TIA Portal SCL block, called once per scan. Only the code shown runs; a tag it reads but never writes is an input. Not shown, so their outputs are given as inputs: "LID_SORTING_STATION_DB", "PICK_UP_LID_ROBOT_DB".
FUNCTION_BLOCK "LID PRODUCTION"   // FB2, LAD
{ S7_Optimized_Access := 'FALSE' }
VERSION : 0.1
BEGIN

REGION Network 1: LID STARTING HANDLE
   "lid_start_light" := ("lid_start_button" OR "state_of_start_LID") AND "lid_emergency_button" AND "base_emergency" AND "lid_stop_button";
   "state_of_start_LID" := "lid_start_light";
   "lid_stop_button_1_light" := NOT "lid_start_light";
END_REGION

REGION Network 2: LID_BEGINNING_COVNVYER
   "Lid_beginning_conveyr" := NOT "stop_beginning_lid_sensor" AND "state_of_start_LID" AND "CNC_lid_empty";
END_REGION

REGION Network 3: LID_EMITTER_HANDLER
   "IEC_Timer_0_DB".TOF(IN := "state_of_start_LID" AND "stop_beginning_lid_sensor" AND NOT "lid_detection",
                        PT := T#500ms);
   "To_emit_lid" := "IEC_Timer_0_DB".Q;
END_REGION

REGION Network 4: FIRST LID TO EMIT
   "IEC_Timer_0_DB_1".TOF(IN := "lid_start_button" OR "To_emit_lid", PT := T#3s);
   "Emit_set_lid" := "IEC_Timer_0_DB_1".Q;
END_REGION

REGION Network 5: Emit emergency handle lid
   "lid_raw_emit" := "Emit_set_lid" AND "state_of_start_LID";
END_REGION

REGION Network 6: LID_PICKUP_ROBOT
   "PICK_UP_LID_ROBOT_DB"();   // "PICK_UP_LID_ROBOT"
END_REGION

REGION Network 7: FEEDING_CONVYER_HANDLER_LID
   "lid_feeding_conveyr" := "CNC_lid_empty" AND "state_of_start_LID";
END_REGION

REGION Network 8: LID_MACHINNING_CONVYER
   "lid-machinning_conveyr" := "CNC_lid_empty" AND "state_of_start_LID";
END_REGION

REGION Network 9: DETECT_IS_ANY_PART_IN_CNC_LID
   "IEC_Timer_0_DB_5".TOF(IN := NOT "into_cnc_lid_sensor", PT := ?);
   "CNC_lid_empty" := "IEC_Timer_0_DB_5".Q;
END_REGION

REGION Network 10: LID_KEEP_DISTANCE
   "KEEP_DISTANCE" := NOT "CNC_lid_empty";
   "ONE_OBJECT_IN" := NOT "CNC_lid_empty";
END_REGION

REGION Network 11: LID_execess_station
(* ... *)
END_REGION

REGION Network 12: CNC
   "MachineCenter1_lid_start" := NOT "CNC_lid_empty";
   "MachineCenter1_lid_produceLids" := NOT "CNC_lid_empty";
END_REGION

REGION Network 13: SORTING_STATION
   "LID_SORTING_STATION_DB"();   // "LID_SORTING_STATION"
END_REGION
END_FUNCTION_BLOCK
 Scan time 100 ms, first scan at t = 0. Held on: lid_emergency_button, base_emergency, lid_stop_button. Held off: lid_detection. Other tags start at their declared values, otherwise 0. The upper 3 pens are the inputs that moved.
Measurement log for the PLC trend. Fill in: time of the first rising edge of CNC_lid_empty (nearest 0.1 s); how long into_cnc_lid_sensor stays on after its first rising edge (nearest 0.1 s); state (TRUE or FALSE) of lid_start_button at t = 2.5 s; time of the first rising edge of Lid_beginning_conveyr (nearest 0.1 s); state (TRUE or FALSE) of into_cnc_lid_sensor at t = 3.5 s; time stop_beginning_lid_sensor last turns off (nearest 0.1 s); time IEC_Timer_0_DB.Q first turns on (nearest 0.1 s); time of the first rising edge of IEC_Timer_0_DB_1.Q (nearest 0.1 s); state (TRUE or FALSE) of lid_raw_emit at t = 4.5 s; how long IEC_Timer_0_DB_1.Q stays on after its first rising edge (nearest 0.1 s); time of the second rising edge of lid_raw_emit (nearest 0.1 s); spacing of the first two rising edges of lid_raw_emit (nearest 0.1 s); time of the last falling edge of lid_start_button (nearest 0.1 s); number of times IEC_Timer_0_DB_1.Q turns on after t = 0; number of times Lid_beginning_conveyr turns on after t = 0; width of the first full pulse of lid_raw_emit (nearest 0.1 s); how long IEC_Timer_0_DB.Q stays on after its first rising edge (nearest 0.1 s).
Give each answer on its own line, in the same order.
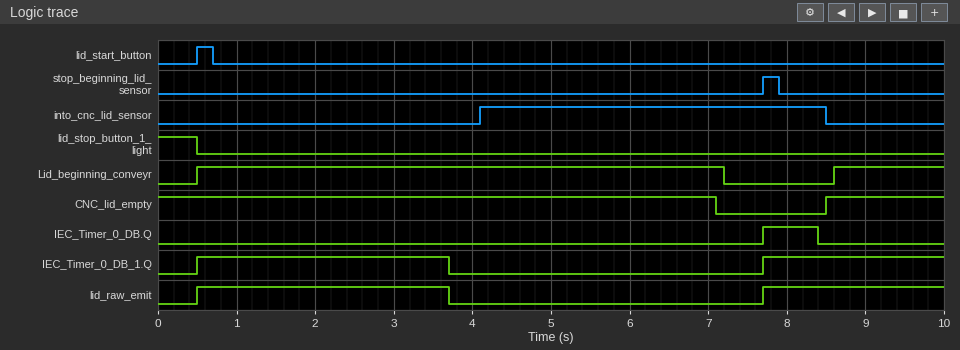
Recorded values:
8.5 s
4.4 s
FALSE
0.5 s
FALSE
7.9 s
7.7 s
0.5 s
FALSE
3.2 s
7.7 s
7.2 s
0.7 s
2
2
3.2 s
0.7 s
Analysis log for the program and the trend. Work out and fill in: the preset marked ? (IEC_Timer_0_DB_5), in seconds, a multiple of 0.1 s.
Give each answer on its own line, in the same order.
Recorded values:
3.0 s
